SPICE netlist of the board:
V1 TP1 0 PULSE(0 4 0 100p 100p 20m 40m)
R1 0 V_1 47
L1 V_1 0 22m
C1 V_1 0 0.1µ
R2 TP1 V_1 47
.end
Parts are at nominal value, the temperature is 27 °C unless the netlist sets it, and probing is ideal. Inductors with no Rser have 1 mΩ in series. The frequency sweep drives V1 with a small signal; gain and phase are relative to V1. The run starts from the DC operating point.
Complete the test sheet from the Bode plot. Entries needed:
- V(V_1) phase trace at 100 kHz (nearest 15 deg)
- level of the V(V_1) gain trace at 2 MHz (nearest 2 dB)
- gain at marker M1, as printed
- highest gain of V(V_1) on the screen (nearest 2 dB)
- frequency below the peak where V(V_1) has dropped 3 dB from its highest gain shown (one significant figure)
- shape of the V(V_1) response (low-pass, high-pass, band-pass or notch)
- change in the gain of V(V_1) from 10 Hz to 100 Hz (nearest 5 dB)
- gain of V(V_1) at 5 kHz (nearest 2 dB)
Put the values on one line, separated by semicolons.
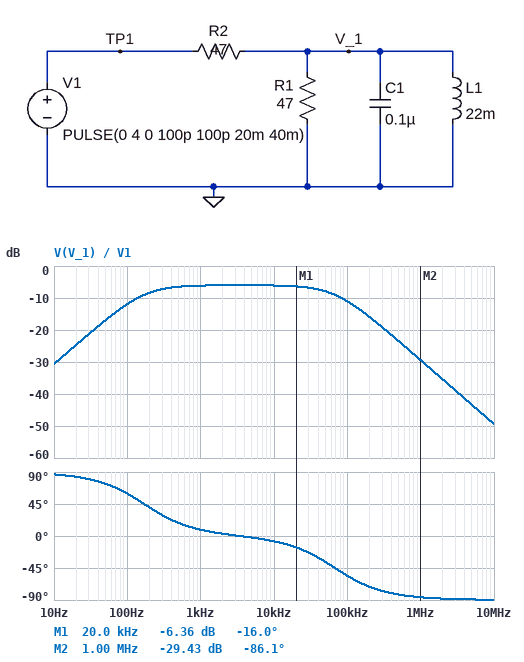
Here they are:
-60 deg; -36 dB; -6.36 dB; -6 dB; 200 Hz; band-pass; 20 dB; -6 dB
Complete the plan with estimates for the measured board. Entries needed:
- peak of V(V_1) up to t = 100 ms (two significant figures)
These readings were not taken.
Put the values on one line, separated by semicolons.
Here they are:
2.0 V
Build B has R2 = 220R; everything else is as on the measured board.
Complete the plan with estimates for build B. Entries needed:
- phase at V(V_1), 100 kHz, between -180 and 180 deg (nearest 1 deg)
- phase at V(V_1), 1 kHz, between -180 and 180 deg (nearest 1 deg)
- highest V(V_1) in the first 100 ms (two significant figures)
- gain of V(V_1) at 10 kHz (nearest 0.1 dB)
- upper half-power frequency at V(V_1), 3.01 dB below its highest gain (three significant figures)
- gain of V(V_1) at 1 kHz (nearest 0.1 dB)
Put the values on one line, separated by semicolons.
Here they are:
-68 deg; 14 deg; 690 mV; -15.3 dB; 41.4 kHz; -15.4 dB
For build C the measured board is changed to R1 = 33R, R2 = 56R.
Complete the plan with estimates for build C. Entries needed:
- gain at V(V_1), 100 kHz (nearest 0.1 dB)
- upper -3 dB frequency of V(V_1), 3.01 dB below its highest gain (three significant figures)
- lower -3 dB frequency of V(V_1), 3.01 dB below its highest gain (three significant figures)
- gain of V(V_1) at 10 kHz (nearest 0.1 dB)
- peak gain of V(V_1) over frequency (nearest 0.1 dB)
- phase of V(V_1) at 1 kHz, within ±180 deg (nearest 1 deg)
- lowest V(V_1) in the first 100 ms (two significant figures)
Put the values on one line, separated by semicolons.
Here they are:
-12.9 dB; 76.8 kHz; 150 Hz; -8.7 dB; -8.6 dB; 8 deg; -1.5 V
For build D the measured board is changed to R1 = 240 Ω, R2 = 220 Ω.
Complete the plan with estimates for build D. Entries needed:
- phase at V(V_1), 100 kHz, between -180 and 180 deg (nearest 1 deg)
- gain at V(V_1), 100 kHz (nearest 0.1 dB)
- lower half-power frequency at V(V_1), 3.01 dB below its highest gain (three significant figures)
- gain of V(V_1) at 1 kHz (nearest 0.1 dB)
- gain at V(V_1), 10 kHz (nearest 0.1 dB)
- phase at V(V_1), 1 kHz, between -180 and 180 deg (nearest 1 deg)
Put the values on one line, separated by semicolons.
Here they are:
-82 deg; -22.9 dB; 786 Hz; -7.6 dB; -7.1 dB; 37 deg
